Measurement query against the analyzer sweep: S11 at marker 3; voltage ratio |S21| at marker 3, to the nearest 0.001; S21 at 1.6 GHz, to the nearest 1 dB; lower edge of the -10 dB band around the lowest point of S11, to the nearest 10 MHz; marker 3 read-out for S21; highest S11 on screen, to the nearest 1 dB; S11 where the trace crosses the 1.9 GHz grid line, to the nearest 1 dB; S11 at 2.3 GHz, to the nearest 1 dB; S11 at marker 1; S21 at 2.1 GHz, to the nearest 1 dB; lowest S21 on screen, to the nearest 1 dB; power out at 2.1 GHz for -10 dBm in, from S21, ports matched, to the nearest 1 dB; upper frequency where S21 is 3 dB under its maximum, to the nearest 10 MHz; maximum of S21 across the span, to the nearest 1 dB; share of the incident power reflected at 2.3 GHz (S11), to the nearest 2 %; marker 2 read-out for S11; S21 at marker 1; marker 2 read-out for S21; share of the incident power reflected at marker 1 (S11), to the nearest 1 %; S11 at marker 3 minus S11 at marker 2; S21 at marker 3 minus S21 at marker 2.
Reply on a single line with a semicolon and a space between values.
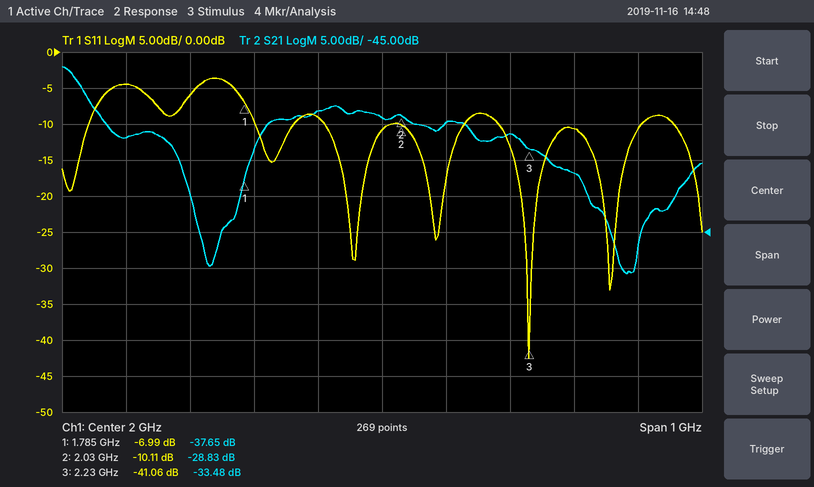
-41.06 dB; 0.021; -32 dB; 2.18 GHz; -33.48 dB; -4 dB; -9 dB; -11 dB; -6.99 dB; -30 dB; -51 dB; -40 dBm; 1.53 GHz; -22 dB; 8 %; -10.11 dB; -37.65 dB; -28.83 dB; 20 %; -30.95 dB; -4.65 dB
